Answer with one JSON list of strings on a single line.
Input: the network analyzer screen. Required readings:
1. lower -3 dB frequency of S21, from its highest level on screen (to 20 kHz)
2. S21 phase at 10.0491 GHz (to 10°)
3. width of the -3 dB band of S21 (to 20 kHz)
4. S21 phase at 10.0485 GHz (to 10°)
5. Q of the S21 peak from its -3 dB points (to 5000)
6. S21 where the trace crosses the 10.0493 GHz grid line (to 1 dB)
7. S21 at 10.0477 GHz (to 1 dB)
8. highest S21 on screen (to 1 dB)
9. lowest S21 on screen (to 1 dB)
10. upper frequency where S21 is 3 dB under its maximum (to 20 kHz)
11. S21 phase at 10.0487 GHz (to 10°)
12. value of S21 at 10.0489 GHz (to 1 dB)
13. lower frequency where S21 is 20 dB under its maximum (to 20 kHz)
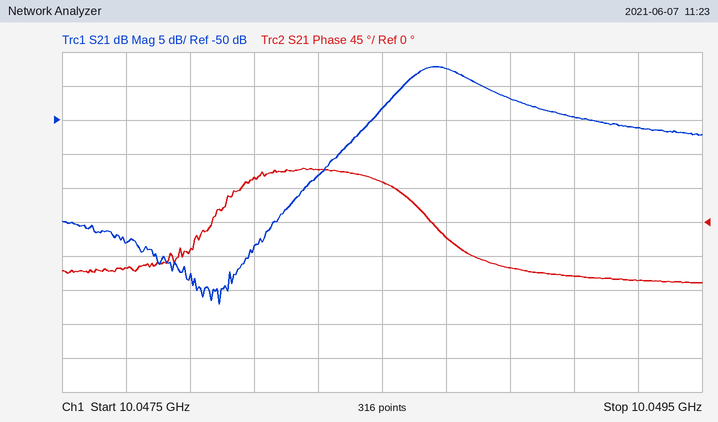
["10.04856 GHz", "-70°", "260 kHz", "50°", "40000", "-51 dB", "-68 dB", "-42 dB", "-77 dB", "10.04882 GHz", "-20°", "-47 dB", "10.04822 GHz"]
